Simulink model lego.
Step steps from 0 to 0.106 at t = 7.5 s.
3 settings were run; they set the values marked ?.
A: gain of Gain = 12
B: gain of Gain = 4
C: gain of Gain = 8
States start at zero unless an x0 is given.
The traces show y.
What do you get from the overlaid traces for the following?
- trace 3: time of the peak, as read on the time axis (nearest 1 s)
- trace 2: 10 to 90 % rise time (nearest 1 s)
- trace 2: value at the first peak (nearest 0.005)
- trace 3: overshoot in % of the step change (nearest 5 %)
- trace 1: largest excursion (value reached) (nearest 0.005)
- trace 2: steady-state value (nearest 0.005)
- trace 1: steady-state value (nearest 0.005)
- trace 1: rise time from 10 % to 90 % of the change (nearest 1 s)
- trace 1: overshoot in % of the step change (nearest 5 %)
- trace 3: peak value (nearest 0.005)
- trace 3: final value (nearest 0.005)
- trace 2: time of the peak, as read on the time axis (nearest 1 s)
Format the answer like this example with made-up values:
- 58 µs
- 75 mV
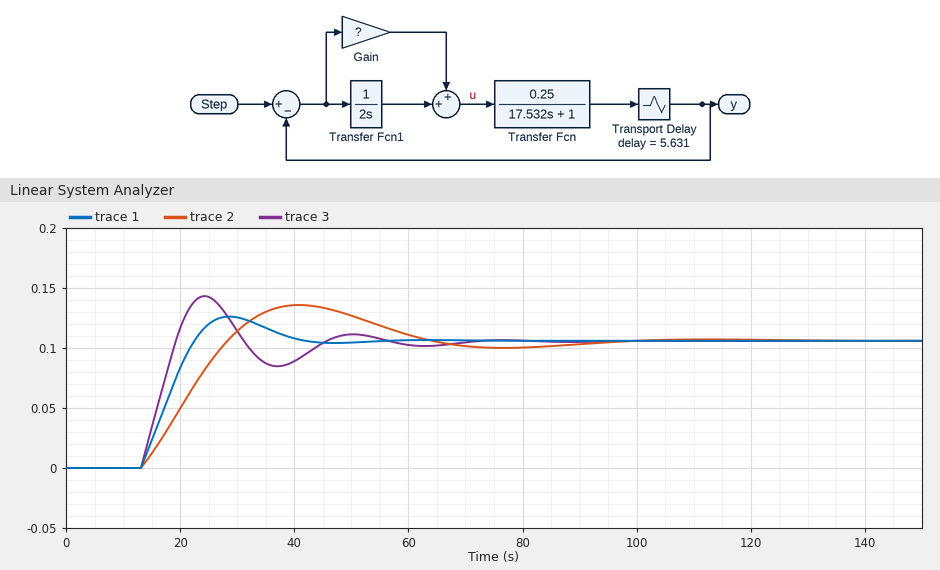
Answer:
- 24 s
- 12 s
- 0.135
- 35 %
- 0.125
- 0.105
- 0.105
- 7 s
- 20 %
- 0.145
- 0.105
- 41 s
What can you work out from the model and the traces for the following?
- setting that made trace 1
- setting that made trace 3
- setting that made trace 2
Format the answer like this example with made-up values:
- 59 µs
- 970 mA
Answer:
- C
- A
- B
